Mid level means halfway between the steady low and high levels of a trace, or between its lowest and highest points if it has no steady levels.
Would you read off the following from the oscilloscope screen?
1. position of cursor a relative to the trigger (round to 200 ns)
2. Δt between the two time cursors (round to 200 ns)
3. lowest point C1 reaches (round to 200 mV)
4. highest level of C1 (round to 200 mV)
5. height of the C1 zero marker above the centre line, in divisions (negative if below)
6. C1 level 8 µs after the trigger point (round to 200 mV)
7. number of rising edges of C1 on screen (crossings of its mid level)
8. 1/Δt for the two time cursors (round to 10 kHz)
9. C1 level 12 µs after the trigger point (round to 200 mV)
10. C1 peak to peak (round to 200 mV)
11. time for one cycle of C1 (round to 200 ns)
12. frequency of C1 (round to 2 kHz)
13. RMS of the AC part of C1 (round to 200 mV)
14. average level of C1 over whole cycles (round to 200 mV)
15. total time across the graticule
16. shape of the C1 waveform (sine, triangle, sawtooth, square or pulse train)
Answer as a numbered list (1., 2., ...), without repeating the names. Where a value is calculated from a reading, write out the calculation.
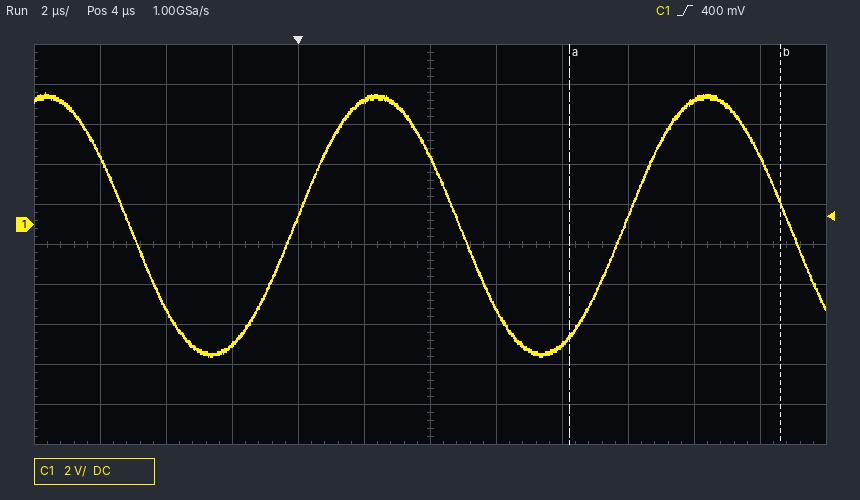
1. +8.2 µs
2. 6.4 µs
3. -6.6 V
4. 6.6 V
5. +0.5 div
6. -6.0 V
7. 2
8. 1 / 6.4 µs ≈ 160 kHz
9. 6.2 V
10. 6.6 V − (-6.6 V) = 13.2 V
11. 10.0 µs
12. 1 / 10.0 µs ≈ 100 kHz
13. 13.2 V / (2√2) ≈ 4.67 V, so 4.6 V to the nearest 200 mV
14. (6.6 V + (-6.6 V)) / 2 ≈ 0.0 V
15. 24 µs
16. sine
